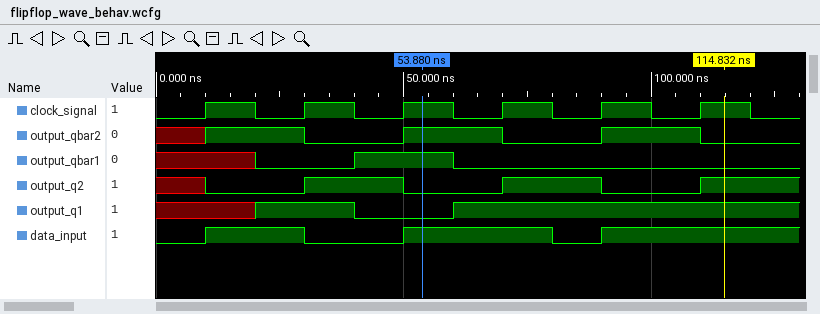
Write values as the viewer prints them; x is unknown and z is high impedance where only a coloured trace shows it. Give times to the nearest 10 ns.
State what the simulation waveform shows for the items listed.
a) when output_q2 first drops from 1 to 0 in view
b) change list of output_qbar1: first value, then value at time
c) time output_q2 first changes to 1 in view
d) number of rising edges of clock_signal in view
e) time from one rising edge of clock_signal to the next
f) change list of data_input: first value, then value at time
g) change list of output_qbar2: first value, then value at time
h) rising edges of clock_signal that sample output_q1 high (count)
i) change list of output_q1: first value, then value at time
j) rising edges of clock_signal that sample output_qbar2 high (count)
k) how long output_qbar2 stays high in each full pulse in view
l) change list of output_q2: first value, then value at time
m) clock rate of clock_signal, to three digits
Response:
50 ns
x, 0 at 20 ns, 1 at 40 ns, 0 at 60 ns
30 ns
6
20 ns
0, 1 at 10 ns, 0 at 30 ns, 1 at 50 ns, 0 at 80 ns, 1 at 90 ns
x, 1 at 10 ns, 0 at 30 ns, 1 at 50 ns, 0 at 70 ns, 1 at 90 ns, 0 at 110 ns
4
x, 1 at 20 ns, 0 at 40 ns, 1 at 60 ns
3
20 ns, 20 ns
x, 0 at 10 ns, 1 at 30 ns, 0 at 50 ns, 1 at 70 ns, 0 at 90 ns, 1 at 110 ns
50.0 MHz
